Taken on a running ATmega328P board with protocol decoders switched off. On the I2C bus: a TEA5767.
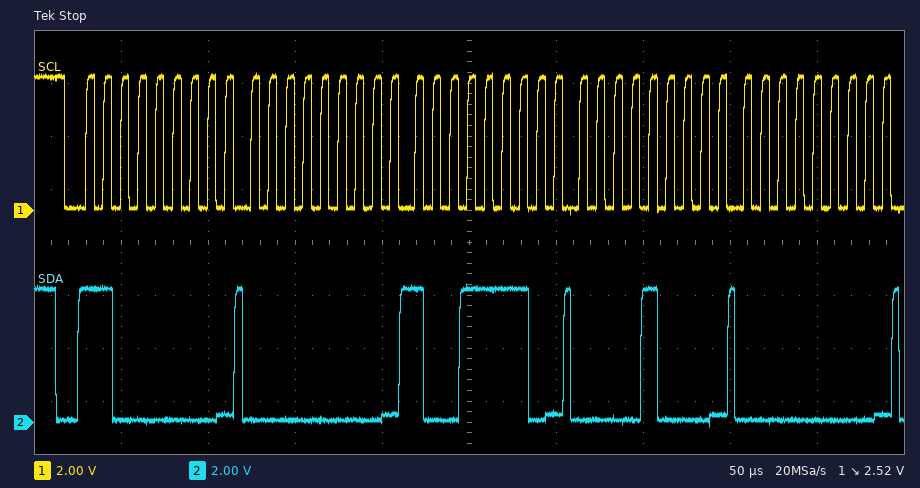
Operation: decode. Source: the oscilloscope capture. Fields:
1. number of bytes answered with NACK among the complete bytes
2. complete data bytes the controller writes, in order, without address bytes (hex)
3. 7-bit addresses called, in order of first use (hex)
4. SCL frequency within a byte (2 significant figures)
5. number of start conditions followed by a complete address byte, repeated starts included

0
00 9E 08 00
0x60
100 kHz
1
